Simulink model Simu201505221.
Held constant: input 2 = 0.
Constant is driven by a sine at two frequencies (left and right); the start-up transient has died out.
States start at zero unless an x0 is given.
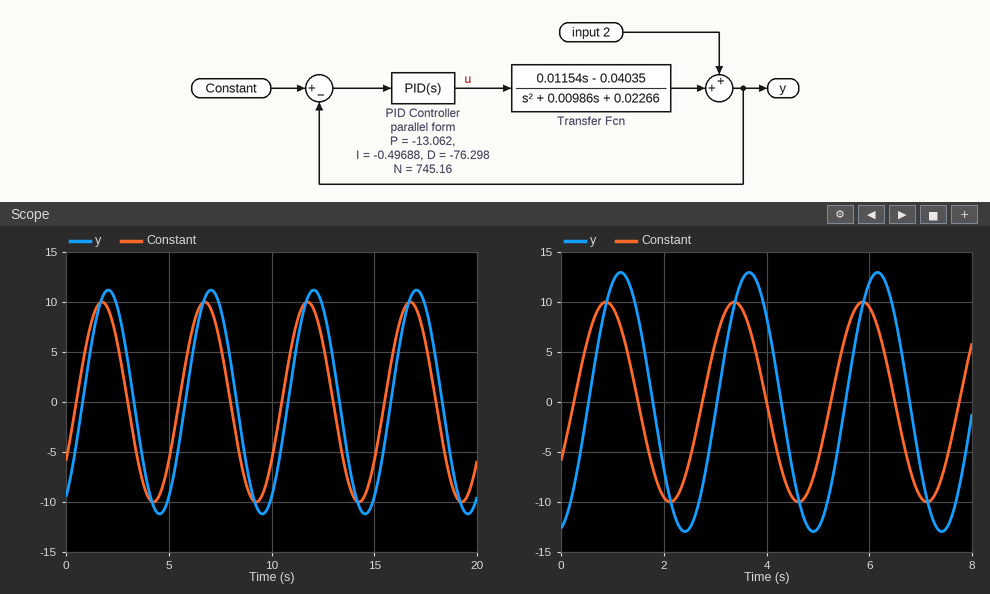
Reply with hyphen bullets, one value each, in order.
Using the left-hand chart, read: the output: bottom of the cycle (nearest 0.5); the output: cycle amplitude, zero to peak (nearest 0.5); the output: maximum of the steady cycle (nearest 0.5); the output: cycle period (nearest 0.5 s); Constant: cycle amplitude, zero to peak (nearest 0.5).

- -11.0
- 11.0
- 11.0
- 5.0 s
- 10.0
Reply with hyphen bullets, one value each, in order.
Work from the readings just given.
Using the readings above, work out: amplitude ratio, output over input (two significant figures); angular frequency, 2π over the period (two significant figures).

- 1.1
- 1.3 rad/s
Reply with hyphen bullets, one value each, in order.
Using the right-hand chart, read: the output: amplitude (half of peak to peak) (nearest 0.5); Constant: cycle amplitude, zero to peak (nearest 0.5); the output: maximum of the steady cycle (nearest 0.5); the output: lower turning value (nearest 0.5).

- 13.0
- 10.0
- 13.0
- -13.0
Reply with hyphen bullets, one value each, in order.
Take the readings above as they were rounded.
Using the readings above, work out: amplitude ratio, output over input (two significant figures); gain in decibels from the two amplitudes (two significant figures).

- 1.3
- 2.3 dB
